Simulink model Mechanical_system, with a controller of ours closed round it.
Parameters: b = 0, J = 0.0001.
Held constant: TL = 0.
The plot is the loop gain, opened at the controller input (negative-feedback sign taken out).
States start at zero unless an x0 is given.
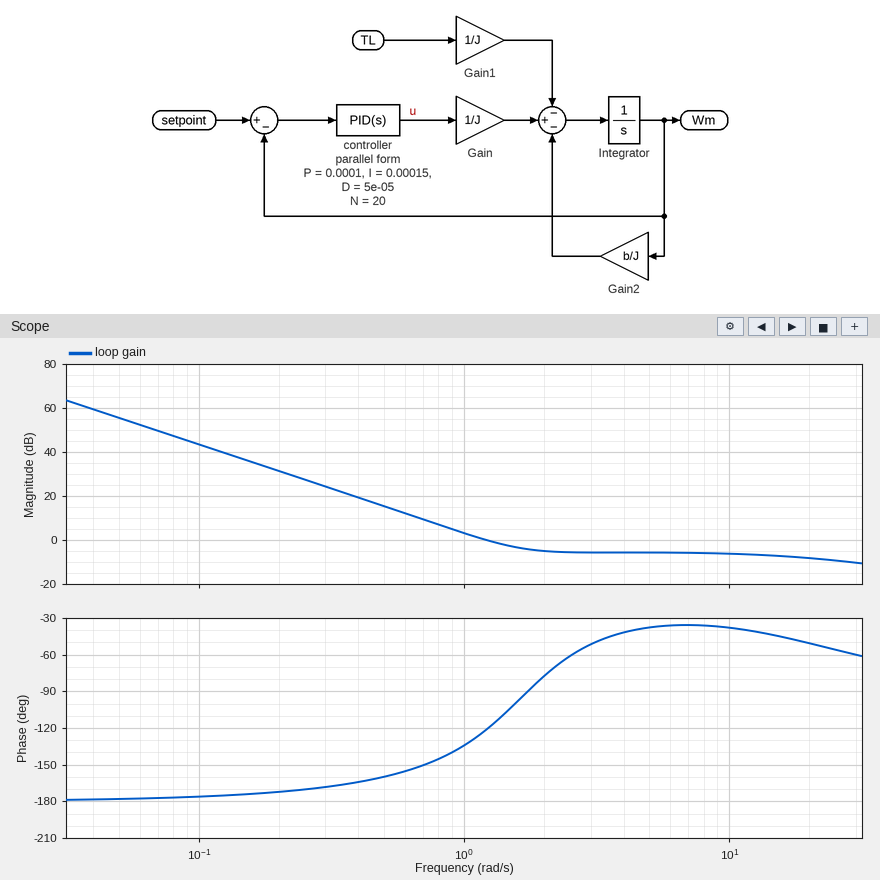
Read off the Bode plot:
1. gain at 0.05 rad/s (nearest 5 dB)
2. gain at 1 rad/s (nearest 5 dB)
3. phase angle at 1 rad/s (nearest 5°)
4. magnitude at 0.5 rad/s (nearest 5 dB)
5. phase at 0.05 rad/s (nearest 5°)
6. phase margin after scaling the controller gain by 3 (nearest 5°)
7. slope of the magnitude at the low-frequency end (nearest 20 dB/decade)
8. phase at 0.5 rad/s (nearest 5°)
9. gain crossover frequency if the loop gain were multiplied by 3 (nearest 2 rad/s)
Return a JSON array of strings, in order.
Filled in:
["55 dB", "5 dB", "-135°", "15 dB", "-180°", "125°", "-40 dB/decade", "-160°", "26 rad/s"]
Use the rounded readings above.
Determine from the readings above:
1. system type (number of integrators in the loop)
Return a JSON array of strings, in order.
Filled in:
["2"]
